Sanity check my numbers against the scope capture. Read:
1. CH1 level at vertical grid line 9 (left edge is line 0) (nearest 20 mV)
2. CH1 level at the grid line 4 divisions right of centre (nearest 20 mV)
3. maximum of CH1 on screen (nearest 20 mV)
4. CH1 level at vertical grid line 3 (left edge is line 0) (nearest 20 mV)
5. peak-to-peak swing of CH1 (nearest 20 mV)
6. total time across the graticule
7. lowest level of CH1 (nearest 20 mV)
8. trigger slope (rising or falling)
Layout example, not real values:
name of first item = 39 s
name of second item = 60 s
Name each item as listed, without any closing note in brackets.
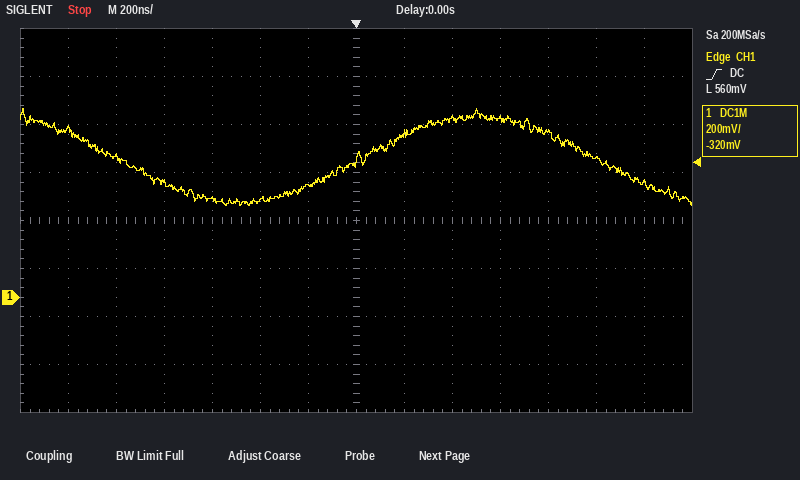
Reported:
CH1 level at vertical grid line 9 (left edge is line 0) = 740 mV
CH1 level at the grid line 4 divisions right of centre = 700 mV
maximum of CH1 on screen = 780 mV
CH1 level at vertical grid line 3 (left edge is line 0) = 480 mV
peak-to-peak swing of CH1 = 400 mV
total time across the graticule = 2.8 µs
lowest level of CH1 = 380 mV
trigger slope = rising
